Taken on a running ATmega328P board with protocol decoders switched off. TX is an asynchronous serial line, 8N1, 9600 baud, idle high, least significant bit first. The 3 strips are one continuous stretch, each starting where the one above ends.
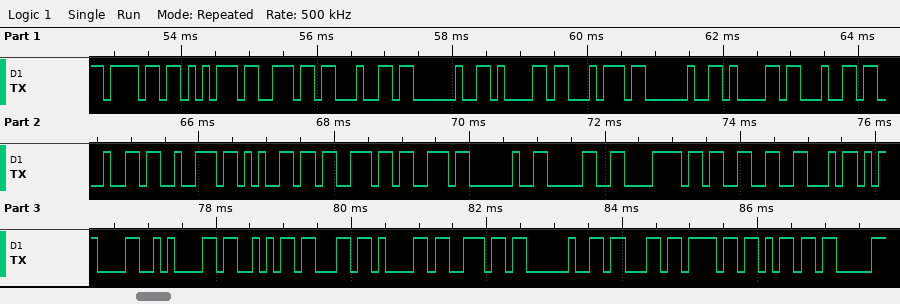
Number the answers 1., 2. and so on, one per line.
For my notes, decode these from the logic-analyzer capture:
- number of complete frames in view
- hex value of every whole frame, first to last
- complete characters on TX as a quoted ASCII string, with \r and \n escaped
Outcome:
1. 30
2. 6F 75 6E 64 20 61 74 20 61 64 64 72 65 73 73 20 30 78 33 46 0D 0A 53 63 61 6E 20 63 6F 6D
3. "ound at address 0x3F\r\nScan com"
